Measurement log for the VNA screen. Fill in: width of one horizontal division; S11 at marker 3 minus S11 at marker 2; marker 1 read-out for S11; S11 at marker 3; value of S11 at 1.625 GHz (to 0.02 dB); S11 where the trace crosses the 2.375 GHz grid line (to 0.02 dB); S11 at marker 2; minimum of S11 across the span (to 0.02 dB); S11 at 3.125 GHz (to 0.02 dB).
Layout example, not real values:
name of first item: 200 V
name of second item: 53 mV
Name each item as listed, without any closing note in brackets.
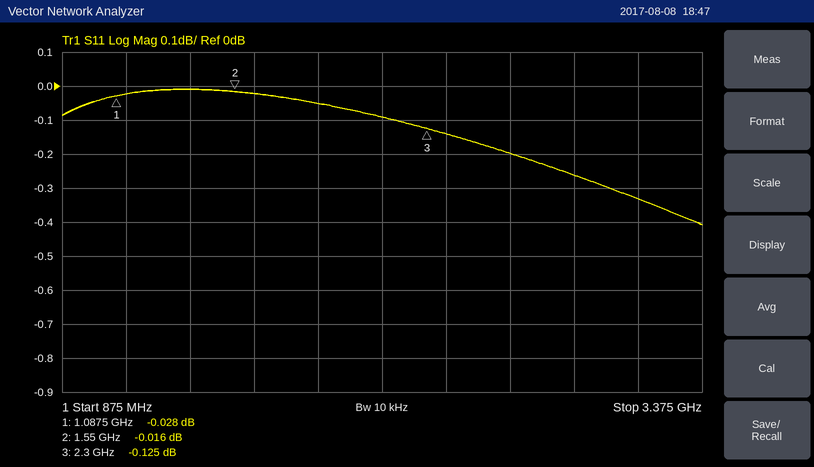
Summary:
width of one horizontal division: 250 MHz
S11 at marker 3 minus S11 at marker 2: -0.109 dB
marker 1 read-out for S11: -0.028 dB
S11 at marker 3: -0.125 dB
value of S11 at 1.625 GHz: -0.02 dB
S11 where the trace crosses the 2.375 GHz grid line: -0.14 dB
S11 at marker 2: -0.016 dB
minimum of S11 across the span: -0.40 dB
S11 at 3.125 GHz: -0.34 dB
